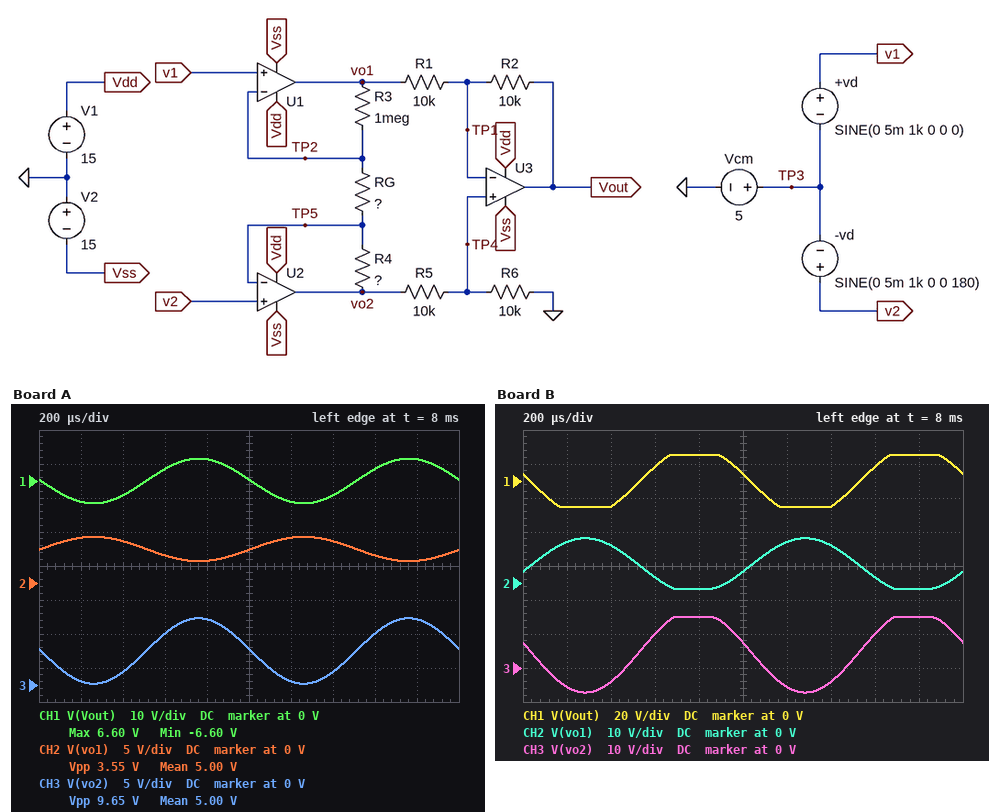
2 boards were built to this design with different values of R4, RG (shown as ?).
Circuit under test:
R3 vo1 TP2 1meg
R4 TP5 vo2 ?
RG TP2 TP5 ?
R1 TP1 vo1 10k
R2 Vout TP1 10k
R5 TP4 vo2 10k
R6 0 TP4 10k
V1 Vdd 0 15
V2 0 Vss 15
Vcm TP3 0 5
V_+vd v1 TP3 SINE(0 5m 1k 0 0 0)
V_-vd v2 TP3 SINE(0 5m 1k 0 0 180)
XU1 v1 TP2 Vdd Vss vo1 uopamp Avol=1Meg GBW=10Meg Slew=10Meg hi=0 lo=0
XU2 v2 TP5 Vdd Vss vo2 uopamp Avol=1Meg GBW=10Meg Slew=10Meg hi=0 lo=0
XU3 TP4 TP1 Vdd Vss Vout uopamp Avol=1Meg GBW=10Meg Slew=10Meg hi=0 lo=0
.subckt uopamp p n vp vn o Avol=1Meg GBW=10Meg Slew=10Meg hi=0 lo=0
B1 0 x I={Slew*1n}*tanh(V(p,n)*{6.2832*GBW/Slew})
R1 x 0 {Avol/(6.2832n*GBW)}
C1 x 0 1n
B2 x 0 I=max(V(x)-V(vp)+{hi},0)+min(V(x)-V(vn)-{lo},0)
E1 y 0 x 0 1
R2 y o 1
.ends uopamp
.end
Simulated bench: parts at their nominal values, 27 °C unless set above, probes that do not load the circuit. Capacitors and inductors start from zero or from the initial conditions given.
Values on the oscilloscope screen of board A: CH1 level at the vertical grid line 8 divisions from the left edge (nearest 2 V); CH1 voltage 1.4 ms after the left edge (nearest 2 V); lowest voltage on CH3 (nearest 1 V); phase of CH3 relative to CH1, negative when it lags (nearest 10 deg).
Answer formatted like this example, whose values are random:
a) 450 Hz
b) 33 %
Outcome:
a) 4 V
b) -4 V
c) 0 V
d) 0 deg
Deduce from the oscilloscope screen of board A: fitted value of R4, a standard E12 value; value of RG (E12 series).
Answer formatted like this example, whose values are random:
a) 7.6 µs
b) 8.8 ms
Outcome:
a) 2.7 MΩ
b) 5.6 kΩ
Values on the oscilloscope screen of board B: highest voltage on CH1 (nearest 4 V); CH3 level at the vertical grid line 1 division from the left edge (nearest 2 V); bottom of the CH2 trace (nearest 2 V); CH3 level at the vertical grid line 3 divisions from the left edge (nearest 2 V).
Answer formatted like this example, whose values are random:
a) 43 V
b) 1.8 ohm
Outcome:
a) 16 V
b) -6 V
c) -2 V
d) 10 V
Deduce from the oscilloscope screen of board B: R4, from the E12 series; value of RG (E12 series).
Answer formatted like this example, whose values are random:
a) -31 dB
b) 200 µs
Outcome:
a) 1.5 MΩ
b) 1.2 kΩ
